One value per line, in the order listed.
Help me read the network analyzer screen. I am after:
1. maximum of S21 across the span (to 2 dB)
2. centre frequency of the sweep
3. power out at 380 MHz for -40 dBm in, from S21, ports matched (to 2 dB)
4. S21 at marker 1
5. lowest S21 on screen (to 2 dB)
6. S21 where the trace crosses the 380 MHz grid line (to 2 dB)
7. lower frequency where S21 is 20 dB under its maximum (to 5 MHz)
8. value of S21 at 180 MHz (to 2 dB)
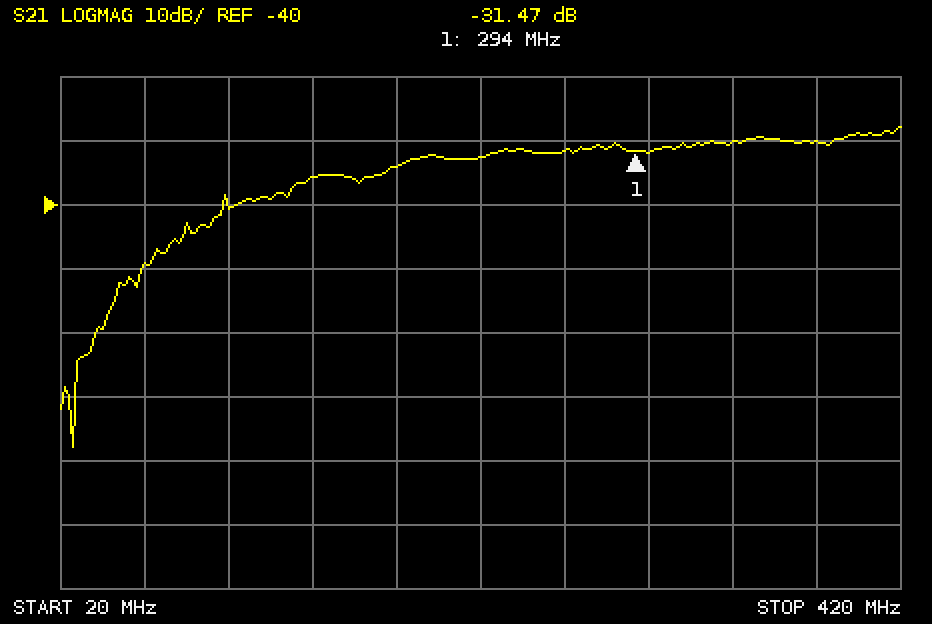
-28 dB
220 MHz
-70 dBm
-31.47 dB
-78 dB
-30 dB
65 MHz
-34 dB
